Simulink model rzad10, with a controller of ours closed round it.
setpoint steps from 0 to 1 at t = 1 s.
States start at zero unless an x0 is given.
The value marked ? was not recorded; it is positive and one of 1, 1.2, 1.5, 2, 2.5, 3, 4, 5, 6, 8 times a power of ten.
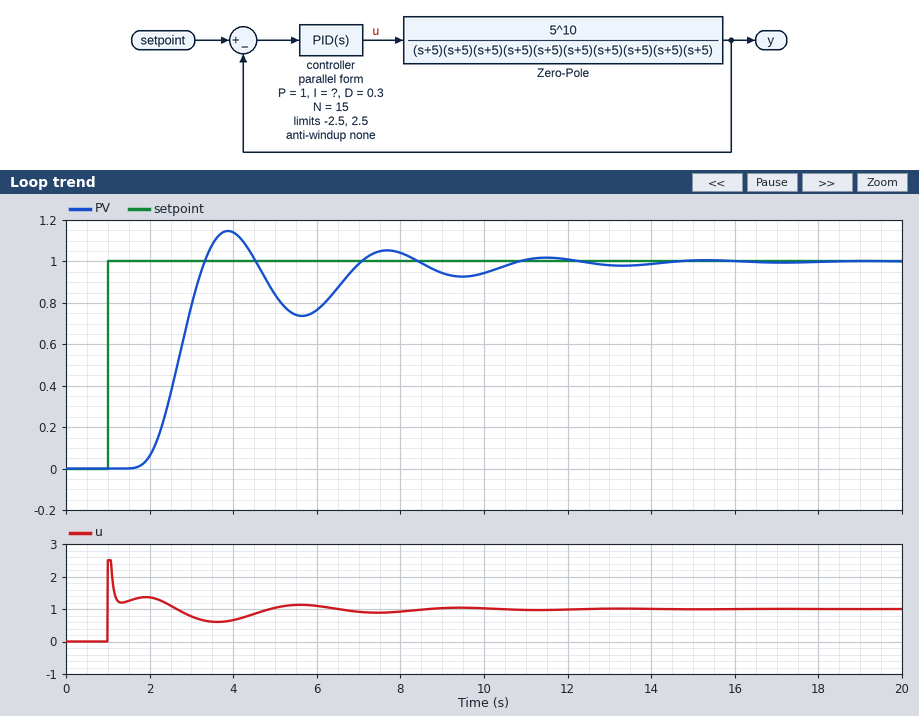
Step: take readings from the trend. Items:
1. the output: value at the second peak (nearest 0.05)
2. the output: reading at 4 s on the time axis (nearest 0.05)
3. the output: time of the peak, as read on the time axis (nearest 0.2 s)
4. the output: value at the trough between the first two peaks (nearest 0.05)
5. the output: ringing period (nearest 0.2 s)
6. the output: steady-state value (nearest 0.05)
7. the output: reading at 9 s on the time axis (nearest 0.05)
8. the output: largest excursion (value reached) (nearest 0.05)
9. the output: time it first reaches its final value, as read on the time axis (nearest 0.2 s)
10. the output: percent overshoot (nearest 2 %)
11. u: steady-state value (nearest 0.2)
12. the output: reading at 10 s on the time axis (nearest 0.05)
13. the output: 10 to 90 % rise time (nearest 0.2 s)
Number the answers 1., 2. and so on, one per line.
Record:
1. 1.05
2. 1.15
3. 3.8 s
4. 0.75
5. 3.8 s
6. 1.00
7. 0.95
8. 1.15
9. 3.4 s
10. 14 %
11. 1.0
12. 0.95
13. 1.0 s
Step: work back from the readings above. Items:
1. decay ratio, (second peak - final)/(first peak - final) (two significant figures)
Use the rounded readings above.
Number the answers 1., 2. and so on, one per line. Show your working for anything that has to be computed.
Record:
1. (1.05 - 1) / (1.15 - 1) = 0.33
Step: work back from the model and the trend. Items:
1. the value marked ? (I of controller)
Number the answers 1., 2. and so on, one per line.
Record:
1. 0.5
